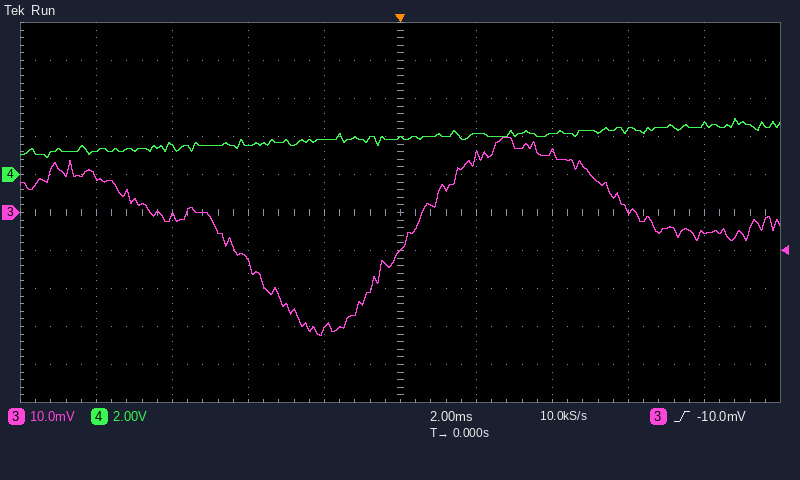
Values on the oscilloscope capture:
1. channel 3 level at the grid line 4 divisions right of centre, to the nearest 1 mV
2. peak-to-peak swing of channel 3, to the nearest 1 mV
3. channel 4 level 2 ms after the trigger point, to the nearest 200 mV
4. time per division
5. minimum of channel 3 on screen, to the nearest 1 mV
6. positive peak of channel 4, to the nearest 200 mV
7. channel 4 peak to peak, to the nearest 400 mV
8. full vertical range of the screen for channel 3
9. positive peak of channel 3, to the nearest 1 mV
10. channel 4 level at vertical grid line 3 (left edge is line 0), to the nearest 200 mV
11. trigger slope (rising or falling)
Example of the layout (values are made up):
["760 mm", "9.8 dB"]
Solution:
["-5 mV", "52 mV", "2.2 V", "2 ms", "-32 mV", "3.0 V", "2.0 V", "100 mV", "20 mV", "1.6 V", "rising"]
